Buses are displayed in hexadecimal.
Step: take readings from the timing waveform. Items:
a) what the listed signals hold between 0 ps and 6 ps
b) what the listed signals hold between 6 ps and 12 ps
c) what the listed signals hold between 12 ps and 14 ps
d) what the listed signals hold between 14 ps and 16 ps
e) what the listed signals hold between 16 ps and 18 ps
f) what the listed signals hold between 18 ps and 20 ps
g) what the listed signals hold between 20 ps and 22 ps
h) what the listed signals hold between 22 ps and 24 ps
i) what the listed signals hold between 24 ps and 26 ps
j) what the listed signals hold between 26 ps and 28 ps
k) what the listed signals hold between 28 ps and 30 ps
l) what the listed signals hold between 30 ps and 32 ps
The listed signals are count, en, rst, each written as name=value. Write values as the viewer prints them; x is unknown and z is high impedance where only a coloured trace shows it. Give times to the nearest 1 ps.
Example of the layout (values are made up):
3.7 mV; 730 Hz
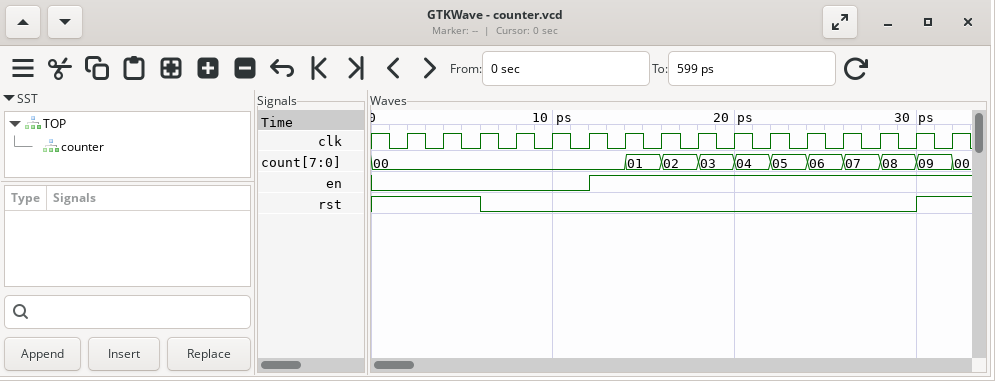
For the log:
count=00, en=0, rst=1; count=00, en=0, rst=0; count=00, en=1, rst=0; count=01, en=1, rst=0; count=02, en=1, rst=0; count=03, en=1, rst=0; count=04, en=1, rst=0; count=05, en=1, rst=0; count=06, en=1, rst=0; count=07, en=1, rst=0; count=08, en=1, rst=0; count=09, en=1, rst=1
